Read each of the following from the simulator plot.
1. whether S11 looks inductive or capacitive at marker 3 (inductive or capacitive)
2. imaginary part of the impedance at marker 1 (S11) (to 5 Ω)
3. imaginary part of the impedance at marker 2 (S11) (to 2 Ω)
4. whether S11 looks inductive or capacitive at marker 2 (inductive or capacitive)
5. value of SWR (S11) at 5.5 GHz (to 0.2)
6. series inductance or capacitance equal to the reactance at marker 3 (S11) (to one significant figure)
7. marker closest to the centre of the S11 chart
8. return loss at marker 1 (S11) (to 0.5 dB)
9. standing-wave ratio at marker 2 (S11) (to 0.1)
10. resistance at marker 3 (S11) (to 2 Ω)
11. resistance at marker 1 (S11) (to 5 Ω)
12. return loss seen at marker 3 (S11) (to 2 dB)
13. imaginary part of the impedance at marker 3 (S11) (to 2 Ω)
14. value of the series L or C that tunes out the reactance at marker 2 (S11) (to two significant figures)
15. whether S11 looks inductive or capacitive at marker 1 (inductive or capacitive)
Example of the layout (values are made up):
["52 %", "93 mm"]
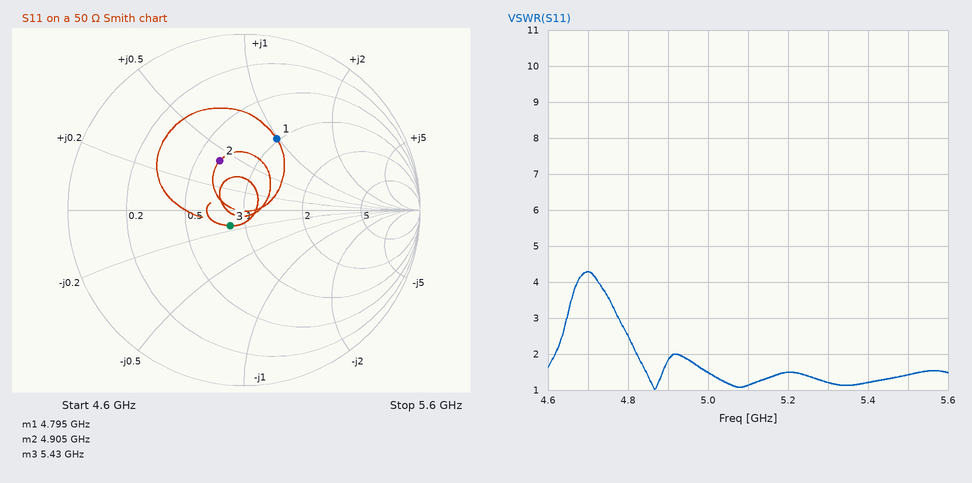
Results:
["capacitive", "+50 Ω", "+20 Ω", "inductive", "1.4", "4 pF", "marker 3", "7.0 dB", "1.9", "42 Ω", "50 Ω", "18 dB", "-8 Ω", "1.6 pF", "inductive"]
